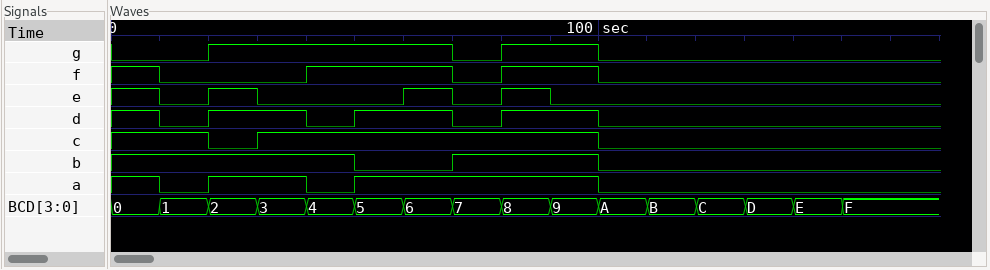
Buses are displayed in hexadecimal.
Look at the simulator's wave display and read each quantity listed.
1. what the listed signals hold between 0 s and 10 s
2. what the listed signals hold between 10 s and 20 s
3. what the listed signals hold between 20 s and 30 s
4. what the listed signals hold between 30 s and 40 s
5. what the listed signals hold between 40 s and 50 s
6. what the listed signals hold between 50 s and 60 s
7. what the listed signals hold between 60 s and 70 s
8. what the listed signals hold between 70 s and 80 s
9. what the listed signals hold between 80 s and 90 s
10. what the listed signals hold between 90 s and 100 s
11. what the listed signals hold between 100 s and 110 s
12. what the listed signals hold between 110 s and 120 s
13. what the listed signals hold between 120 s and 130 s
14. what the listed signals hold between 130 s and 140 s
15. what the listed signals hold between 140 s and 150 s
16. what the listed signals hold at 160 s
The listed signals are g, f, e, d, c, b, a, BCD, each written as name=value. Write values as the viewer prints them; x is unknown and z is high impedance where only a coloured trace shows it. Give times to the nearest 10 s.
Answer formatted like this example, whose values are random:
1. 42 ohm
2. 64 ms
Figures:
1. g=0, f=1, e=1, d=1, c=1, b=1, a=1, BCD=0
2. g=0, f=0, e=0, d=0, c=1, b=1, a=0, BCD=1
3. g=1, f=0, e=1, d=1, c=0, b=1, a=1, BCD=2
4. g=1, f=0, e=0, d=1, c=1, b=1, a=1, BCD=3
5. g=1, f=1, e=0, d=0, c=1, b=1, a=0, BCD=4
6. g=1, f=1, e=0, d=1, c=1, b=0, a=1, BCD=5
7. g=1, f=1, e=1, d=1, c=1, b=0, a=1, BCD=6
8. g=0, f=0, e=0, d=0, c=1, b=1, a=1, BCD=7
9. g=1, f=1, e=1, d=1, c=1, b=1, a=1, BCD=8
10. g=1, f=1, e=0, d=1, c=1, b=1, a=1, BCD=9
11. g=0, f=0, e=0, d=0, c=0, b=0, a=0, BCD=A
12. g=0, f=0, e=0, d=0, c=0, b=0, a=0, BCD=B
13. g=0, f=0, e=0, d=0, c=0, b=0, a=0, BCD=C
14. g=0, f=0, e=0, d=0, c=0, b=0, a=0, BCD=D
15. g=0, f=0, e=0, d=0, c=0, b=0, a=0, BCD=E
16. g=0, f=0, e=0, d=0, c=0, b=0, a=0, BCD=F
